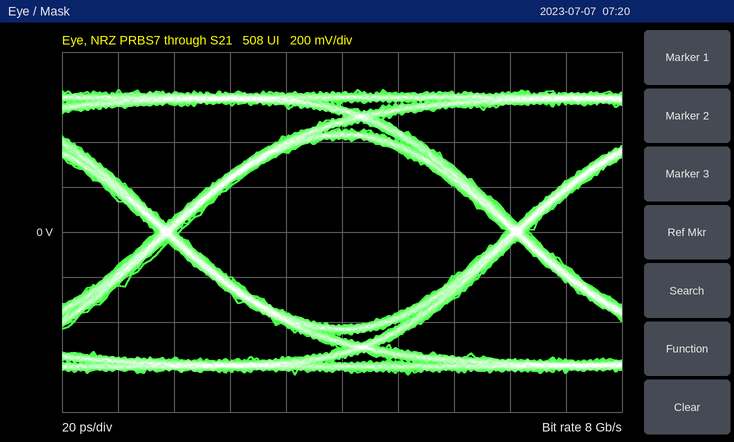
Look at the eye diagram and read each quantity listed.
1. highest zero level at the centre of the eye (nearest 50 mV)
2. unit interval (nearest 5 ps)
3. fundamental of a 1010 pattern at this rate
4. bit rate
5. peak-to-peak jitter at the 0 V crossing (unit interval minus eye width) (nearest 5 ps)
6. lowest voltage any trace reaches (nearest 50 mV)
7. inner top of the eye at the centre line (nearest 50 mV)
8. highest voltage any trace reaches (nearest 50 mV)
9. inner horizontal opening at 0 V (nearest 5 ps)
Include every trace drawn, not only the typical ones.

-400 mV
125 ps
4 GHz
8 Gb/s
10 ps
-650 mV
400 mV
650 mV
115 ps
